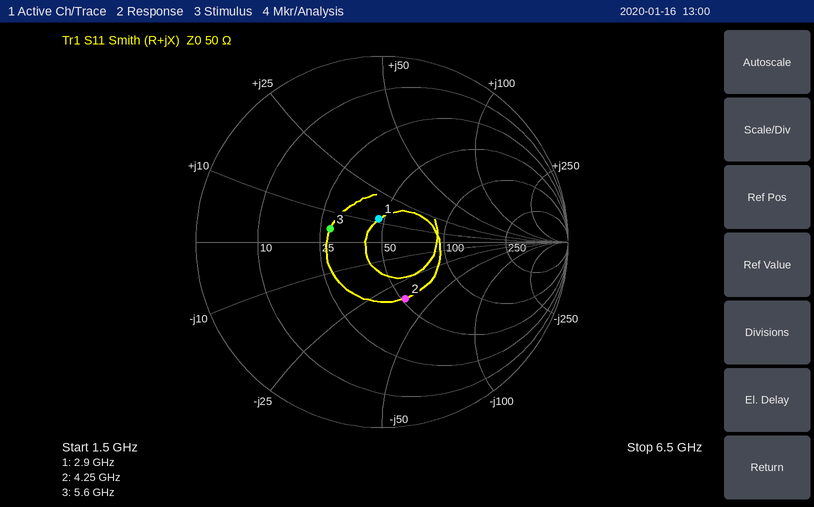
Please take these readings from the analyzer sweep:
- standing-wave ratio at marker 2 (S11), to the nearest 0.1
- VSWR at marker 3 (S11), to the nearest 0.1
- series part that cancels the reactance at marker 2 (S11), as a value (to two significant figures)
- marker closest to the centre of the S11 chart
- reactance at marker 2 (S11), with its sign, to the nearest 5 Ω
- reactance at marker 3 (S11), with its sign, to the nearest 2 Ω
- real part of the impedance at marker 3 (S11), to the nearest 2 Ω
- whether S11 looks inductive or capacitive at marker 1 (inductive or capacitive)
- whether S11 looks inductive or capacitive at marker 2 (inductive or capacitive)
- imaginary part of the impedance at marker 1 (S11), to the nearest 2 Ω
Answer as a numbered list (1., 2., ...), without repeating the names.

1. 2.0
2. 1.8
3. 1.3 nH
4. marker 1
5. -35 Ω
6. +4 Ω
7. 28 Ω
8. inductive
9. capacitive
10. +12 Ω
